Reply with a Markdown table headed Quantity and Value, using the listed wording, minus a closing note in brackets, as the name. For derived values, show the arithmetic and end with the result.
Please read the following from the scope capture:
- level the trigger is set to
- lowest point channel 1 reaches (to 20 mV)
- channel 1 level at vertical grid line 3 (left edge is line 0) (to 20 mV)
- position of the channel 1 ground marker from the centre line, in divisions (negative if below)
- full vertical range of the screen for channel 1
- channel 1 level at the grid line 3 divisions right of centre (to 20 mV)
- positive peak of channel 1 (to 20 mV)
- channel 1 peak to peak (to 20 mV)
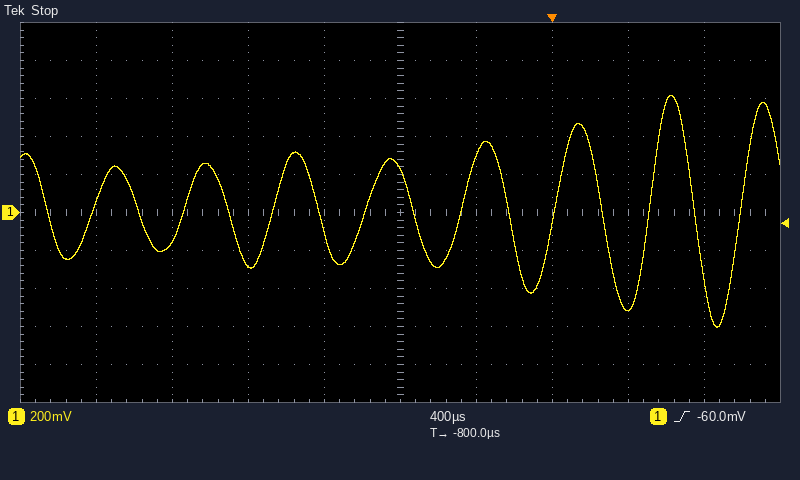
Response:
| Quantity | Value |
|---|---|
| level the trigger is set to | -60.0 mV |
| lowest point channel 1 reaches | -600 mV |
| channel 1 level at vertical grid line 3 (left edge is line 0) | -280 mV |
| position of the channel 1 ground marker from the centre line, in divisions | 0.0 div |
| full vertical range of the screen for channel 1 | 2 V |
| channel 1 level at the grid line 3 divisions right of centre | -500 mV |
| positive peak of channel 1 | 620 mV |
| channel 1 peak to peak | 620 mV − (-600 mV) = 1.22 V |
